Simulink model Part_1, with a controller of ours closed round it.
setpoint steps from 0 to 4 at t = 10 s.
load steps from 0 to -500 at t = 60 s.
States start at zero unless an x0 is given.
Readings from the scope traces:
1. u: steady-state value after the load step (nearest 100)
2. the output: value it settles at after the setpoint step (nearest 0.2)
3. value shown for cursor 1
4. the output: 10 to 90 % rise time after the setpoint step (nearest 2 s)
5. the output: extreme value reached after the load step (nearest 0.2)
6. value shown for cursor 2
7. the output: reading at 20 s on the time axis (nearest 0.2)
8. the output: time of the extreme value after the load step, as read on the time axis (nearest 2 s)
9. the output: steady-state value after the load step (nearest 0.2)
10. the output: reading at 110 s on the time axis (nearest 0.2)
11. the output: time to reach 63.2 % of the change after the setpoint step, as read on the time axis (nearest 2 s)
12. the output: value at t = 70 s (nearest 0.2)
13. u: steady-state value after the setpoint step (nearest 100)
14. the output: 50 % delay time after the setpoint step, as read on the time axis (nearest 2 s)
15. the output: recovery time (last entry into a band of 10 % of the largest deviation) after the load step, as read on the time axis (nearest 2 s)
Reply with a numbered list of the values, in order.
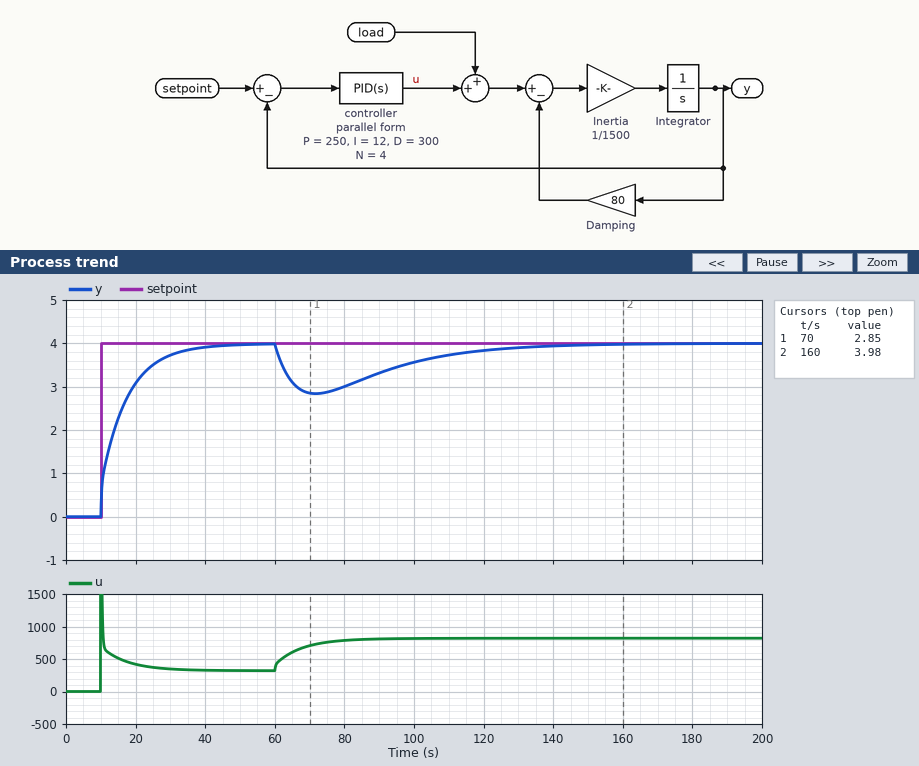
1. 800
2. 4.0
3. 2.85
4. 16 s
5. 2.8
6. 3.98
7. 3.0
8. 72 s
9. 4.0
10. 3.8
11. 16 s
12. 2.8
13. 300
14. 14 s
15. 128 s
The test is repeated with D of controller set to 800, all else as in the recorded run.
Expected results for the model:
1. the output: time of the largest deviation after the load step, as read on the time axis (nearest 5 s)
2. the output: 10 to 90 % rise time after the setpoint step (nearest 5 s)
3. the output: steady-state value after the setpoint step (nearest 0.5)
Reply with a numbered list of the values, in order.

1. 75 s
2. 20 s
3. 4.0
